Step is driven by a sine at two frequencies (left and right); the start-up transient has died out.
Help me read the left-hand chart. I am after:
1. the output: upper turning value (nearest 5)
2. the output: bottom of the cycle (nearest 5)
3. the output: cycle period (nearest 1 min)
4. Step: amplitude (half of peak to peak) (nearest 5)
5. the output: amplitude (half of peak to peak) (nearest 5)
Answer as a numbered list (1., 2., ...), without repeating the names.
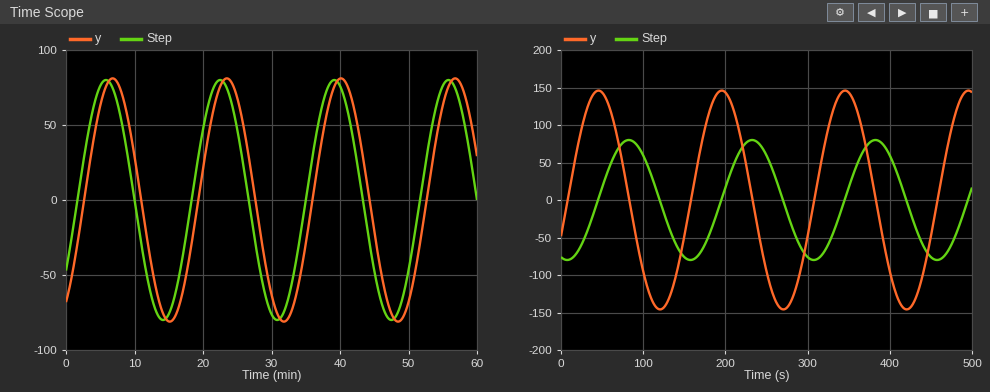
1. 80
2. -80
3. 17 min
4. 80
5. 80
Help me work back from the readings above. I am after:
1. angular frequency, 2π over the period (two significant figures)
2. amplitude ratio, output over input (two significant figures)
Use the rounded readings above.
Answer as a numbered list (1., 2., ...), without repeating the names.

1. 0.37 rad/min
2. 1.0
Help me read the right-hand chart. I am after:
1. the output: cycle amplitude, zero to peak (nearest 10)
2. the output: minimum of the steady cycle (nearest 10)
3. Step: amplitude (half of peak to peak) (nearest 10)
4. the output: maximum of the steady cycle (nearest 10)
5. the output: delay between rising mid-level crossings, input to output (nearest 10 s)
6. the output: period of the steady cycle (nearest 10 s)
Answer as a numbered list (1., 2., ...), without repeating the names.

1. 150
2. -150
3. 80
4. 150
5. 110 s
6. 150 s
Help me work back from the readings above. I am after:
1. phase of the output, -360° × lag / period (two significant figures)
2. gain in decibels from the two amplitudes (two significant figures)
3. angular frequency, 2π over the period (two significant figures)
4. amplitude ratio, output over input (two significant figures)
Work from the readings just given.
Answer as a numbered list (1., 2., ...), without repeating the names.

1. -260°
2. 5.5 dB
3. 0.042 rad/s
4. 1.9
